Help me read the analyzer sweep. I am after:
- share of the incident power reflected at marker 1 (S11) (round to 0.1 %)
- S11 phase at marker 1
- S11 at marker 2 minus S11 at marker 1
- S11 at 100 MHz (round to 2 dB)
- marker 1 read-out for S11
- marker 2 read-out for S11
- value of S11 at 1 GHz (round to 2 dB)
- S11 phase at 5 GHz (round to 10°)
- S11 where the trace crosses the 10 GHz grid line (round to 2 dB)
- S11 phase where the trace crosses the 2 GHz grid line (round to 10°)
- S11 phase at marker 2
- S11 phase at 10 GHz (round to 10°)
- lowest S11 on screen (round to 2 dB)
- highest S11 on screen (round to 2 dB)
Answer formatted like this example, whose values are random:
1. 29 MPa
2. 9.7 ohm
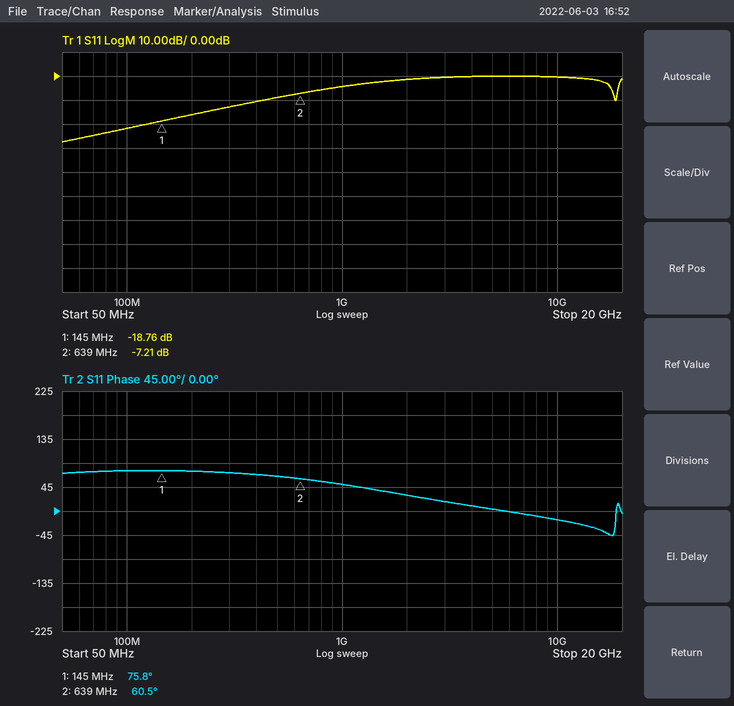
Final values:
1. 1.3 %
2. 75.8°
3. 11.55 dB
4. -22 dB
5. -18.76 dB
6. -7.21 dB
7. -4 dB
8. 0°
9. 0 dB
10. 30°
11. 60.5°
12. -20°
13. -28 dB
14. 0 dB
